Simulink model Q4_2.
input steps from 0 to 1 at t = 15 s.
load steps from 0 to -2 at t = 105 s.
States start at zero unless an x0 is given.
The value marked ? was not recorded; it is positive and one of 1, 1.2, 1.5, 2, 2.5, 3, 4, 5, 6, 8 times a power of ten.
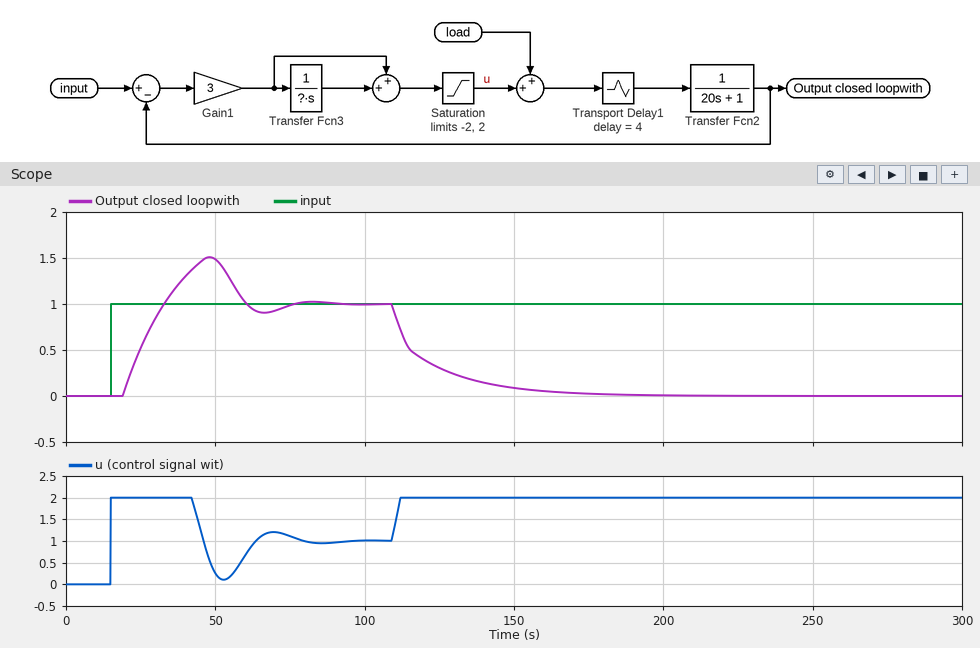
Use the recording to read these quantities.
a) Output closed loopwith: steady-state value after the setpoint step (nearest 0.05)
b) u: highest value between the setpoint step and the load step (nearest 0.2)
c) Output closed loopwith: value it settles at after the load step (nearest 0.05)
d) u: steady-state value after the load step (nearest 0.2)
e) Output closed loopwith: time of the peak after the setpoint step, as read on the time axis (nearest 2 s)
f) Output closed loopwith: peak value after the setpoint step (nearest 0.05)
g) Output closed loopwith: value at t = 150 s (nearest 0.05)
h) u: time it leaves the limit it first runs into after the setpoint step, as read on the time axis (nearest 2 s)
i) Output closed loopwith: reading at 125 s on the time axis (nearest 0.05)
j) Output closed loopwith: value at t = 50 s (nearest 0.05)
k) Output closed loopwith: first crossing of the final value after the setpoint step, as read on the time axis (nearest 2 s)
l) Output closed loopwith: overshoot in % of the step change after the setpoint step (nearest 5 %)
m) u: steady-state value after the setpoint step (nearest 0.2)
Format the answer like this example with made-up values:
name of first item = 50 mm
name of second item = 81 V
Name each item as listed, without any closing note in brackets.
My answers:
Output closed loopwith: steady-state value after the setpoint step = 1.00
u: highest value between the setpoint step and the load step = 2.0
Output closed loopwith: value it settles at after the load step = 0.00
u: steady-state value after the load step = 2.0
Output closed loopwith: time of the peak after the setpoint step, as read on the time axis = 48 s
Output closed loopwith: peak value after the setpoint step = 1.50
Output closed loopwith: value at t = 150 s = 0.10
u: time it leaves the limit it first runs into after the setpoint step, as read on the time axis = 42 s
Output closed loopwith: reading at 125 s on the time axis = 0.30
Output closed loopwith: value at t = 50 s = 1.50
Output closed loopwith: first crossing of the final value after the setpoint step, as read on the time axis = 32 s
Output closed loopwith: overshoot in % of the step change after the setpoint step = 50 %
u: steady-state value after the setpoint step = 1.0
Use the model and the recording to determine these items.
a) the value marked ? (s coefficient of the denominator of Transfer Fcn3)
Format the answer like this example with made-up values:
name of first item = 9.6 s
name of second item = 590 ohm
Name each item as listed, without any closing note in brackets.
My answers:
the value marked ? = 8
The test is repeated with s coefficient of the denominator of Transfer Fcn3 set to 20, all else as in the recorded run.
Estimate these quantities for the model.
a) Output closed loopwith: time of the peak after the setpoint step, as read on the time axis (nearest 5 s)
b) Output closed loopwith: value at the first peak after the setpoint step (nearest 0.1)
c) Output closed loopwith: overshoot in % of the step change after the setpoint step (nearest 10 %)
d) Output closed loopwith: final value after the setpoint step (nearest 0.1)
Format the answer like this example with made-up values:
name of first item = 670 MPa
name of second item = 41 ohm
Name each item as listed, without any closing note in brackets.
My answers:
Output closed loopwith: time of the peak after the setpoint step, as read on the time axis = 40 s
Output closed loopwith: value at the first peak after the setpoint step = 1.2
Output closed loopwith: overshoot in % of the step change after the setpoint step = 20 %
Output closed loopwith: final value after the setpoint step = 1.0
